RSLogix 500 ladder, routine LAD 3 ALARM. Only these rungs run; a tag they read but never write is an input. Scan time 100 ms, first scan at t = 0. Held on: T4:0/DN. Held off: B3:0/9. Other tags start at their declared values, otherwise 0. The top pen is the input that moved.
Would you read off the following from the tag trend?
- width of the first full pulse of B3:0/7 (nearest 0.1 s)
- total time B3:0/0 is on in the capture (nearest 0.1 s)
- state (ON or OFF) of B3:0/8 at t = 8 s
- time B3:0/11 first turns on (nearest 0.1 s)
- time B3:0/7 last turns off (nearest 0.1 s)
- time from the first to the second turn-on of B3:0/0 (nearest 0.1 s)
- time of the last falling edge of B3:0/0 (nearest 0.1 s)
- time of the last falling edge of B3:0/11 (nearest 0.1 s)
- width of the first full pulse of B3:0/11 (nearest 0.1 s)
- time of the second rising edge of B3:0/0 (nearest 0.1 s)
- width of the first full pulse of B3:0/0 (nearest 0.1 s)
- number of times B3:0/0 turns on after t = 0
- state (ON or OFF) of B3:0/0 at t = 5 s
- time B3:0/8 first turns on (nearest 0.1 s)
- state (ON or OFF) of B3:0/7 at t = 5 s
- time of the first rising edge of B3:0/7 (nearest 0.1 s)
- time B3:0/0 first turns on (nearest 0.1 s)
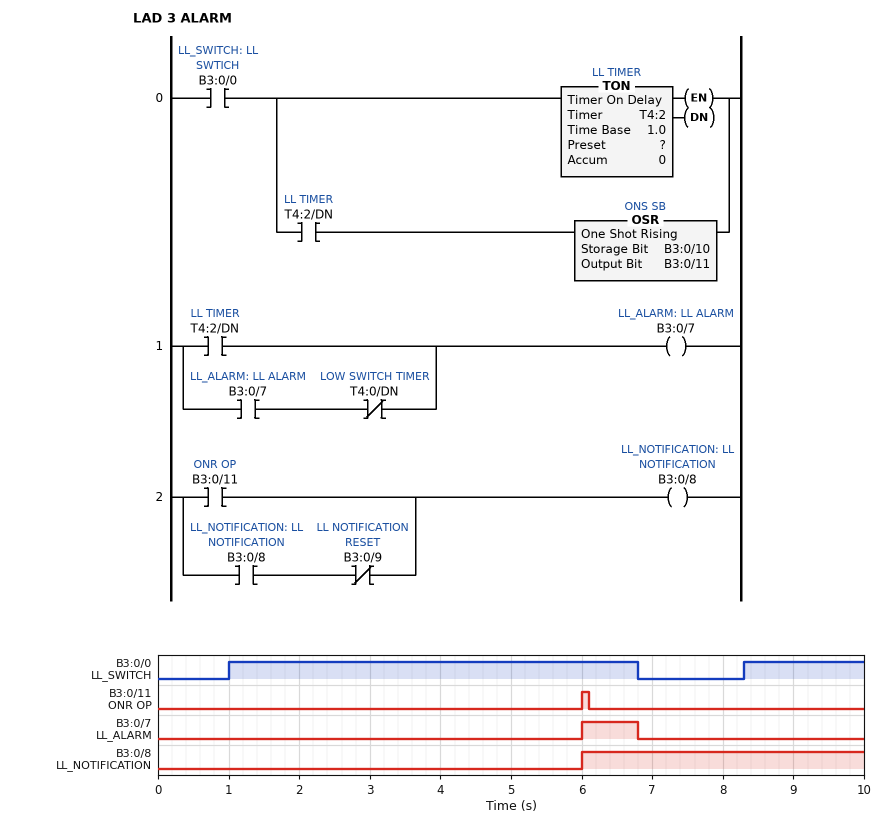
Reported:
0.8 s
7.5 s
ON
6.0 s
6.8 s
7.3 s
6.8 s
6.1 s
0.1 s
8.3 s
5.8 s
2
ON
6.0 s
OFF
6.0 s
1.0 s
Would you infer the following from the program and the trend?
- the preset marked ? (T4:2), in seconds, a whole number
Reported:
5 s
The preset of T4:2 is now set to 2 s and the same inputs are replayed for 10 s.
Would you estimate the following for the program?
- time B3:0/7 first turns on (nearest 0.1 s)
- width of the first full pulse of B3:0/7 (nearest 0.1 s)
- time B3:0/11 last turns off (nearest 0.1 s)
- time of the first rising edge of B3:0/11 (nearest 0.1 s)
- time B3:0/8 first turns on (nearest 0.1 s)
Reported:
3.0 s
3.8 s
3.1 s
3.0 s
3.0 s
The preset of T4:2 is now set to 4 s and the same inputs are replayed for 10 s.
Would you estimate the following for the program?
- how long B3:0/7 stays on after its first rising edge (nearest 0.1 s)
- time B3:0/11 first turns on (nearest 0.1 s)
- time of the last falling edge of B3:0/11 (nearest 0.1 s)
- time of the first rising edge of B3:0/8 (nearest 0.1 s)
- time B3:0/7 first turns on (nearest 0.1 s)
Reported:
1.8 s
5.0 s
5.1 s
5.0 s
5.0 s
